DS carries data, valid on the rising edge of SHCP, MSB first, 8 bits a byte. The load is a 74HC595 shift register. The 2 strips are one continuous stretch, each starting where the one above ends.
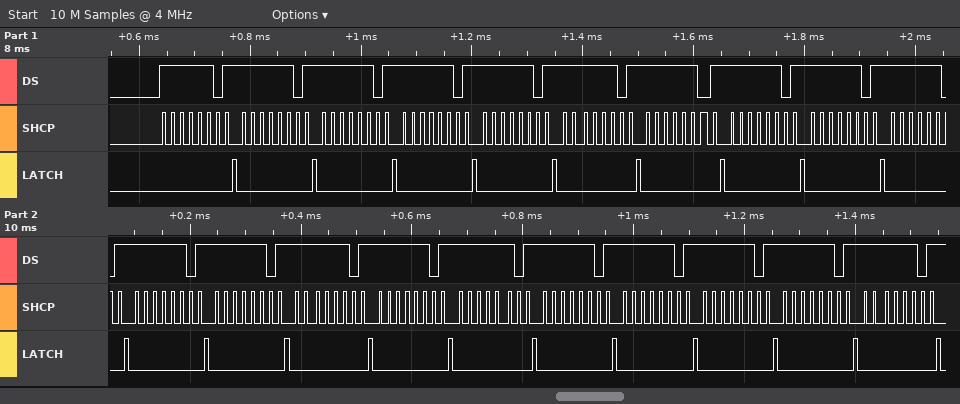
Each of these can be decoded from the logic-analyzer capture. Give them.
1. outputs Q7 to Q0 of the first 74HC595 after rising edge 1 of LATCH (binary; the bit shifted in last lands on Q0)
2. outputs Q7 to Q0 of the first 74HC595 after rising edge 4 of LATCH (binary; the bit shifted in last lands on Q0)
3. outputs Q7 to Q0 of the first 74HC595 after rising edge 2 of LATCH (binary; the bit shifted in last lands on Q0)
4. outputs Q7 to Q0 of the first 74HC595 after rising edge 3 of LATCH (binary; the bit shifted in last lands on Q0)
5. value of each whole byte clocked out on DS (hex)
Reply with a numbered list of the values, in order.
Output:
1. 11111101
2. 11111101
3. 11111101
4. 11111101
5. 0xFD 0xFD 0xFD 0xFD 0xFD 0xFD 0xFD 0xFD 0xFD 0xFD 0xFD 0xFD 0xFD 0xFD 0xFD 0xFD 0xFD 0xFD 0xFD 0xFD
